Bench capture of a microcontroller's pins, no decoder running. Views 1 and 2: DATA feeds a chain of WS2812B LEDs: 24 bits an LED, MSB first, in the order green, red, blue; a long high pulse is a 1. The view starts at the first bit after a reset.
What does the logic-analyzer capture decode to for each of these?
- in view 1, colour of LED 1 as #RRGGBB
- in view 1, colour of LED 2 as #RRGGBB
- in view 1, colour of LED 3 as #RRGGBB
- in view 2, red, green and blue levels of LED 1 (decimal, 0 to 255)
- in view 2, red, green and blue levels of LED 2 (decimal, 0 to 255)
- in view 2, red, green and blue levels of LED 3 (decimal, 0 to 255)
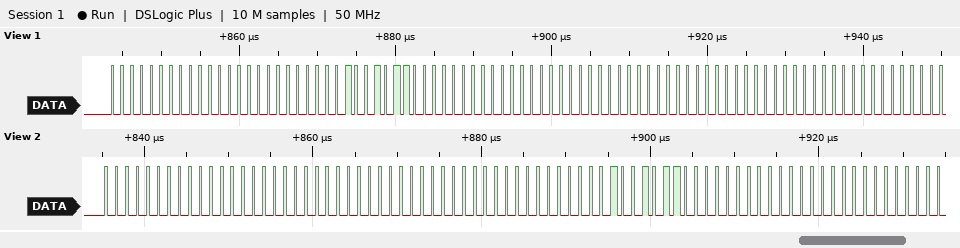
#000000
#009600
#000000
0, 0, 0
0, 0, 0
0, 150, 0
